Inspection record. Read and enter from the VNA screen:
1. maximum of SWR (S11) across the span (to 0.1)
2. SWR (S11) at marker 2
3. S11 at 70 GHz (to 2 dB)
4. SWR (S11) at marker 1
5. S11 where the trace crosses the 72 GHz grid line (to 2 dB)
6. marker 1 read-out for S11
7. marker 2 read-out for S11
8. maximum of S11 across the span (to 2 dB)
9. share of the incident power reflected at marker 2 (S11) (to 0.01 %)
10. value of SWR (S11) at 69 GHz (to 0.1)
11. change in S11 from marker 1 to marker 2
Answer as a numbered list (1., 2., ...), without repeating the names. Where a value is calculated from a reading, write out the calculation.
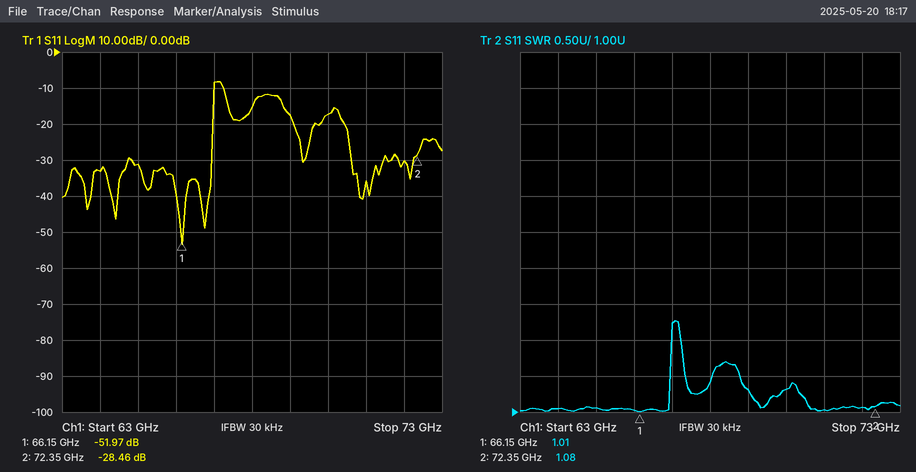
1. 2.3
2. 1.08
3. -18 dB
4. 1.01
5. -30 dB
6. -51.97 dB
7. -28.46 dB
8. -8 dB
9. 10^(-28.46/10) ≈ 0.14 %
10. 1.3
11. -28.46 − (-51.97) = 23.51 dB
